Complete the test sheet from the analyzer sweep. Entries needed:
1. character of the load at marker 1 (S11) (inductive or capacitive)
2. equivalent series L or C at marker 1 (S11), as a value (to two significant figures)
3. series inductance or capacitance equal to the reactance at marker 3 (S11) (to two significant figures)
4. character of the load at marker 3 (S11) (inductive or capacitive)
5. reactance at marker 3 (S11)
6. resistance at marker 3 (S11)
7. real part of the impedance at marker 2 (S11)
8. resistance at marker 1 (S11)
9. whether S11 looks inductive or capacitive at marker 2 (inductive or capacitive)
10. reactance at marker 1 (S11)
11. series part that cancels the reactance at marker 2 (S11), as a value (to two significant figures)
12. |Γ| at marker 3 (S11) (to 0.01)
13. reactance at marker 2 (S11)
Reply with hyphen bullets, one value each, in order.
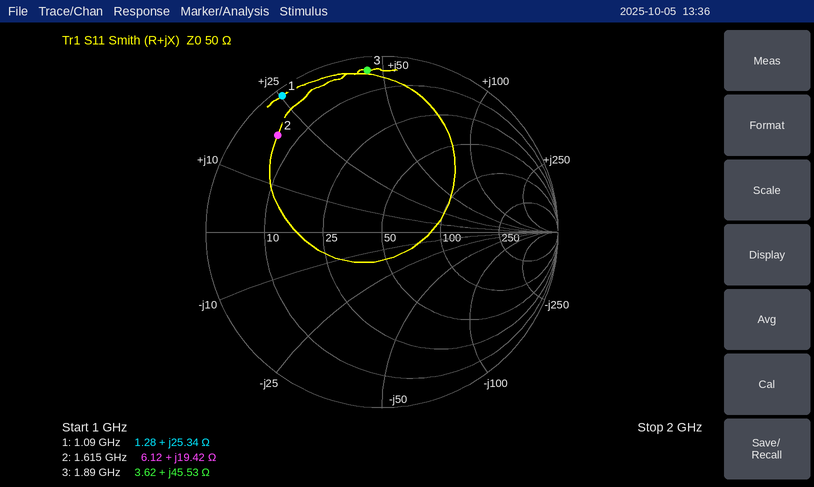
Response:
- inductive
- 3.7 nH
- 3.8 nH
- inductive
- +45.53 Ω
- 3.62 Ω
- 6.12 Ω
- 1.28 Ω
- inductive
- +25.34 Ω
- 5.1 pF
- 0.92
- +19.42 Ω
